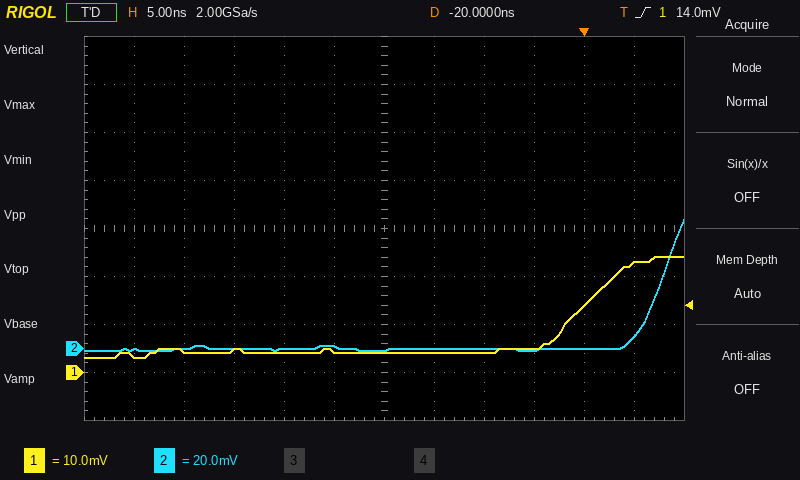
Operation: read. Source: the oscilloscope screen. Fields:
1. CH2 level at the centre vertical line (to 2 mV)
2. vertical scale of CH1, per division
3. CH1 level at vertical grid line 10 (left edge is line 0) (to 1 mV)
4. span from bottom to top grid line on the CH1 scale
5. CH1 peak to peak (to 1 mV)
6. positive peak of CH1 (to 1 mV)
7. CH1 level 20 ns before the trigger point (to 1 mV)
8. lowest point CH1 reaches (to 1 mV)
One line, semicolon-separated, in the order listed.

0 mV; 10 mV; 14 mV; 80 mV; 21 mV; 24 mV; 4 mV; 3 mV
